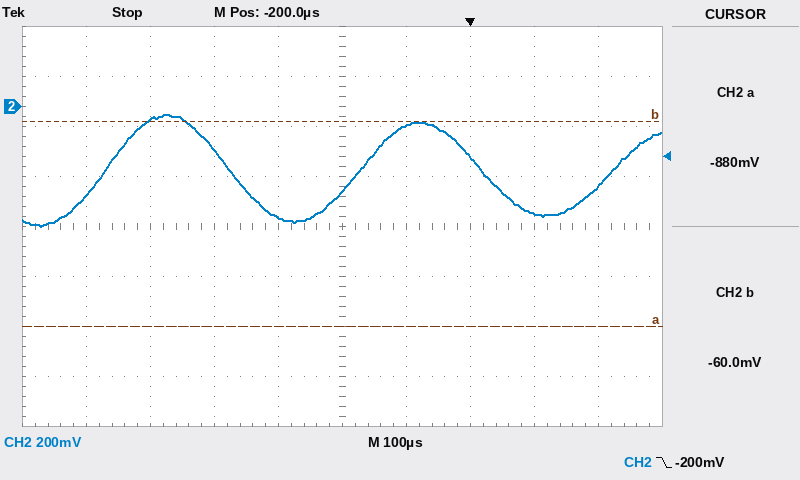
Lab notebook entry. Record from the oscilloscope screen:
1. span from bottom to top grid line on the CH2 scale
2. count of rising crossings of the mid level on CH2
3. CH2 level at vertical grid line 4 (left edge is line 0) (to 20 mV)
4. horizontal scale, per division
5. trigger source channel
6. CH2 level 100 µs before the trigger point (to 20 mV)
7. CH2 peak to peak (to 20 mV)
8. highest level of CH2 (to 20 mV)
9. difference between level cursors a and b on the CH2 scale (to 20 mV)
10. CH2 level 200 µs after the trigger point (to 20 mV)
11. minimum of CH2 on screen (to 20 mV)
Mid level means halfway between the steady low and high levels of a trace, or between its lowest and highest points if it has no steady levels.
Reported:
1.6 V
3
-440 mV
100 µs
CH2
-80 mV
440 mV
-40 mV
820 mV
-320 mV
-480 mV
